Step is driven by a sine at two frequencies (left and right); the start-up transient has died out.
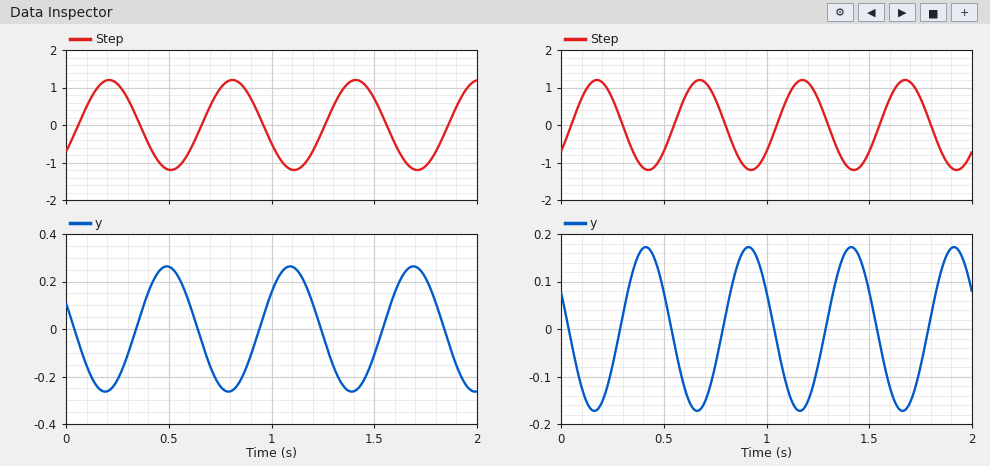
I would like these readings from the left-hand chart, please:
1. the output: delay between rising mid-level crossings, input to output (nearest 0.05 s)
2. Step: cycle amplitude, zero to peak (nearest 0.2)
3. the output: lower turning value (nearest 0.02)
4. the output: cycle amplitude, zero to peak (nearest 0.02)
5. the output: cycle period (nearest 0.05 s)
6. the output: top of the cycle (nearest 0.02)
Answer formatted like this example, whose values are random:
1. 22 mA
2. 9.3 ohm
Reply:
1. 0.30 s
2. 1.2
3. -0.26
4. 0.26
5. 0.60 s
6. 0.26
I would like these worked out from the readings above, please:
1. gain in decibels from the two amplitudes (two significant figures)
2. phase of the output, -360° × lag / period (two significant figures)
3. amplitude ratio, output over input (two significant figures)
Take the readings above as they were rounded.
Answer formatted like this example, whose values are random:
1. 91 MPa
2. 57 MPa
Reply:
1. -13 dB
2. -180°
3. 0.22
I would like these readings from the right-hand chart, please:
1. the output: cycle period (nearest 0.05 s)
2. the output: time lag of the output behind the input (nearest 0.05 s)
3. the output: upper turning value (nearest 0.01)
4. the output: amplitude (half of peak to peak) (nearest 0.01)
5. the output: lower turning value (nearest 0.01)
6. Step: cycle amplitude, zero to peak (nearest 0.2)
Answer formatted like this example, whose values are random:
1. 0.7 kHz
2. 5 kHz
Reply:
1. 0.50 s
2. 0.25 s
3. 0.17
4. 0.17
5. -0.17
6. 1.2
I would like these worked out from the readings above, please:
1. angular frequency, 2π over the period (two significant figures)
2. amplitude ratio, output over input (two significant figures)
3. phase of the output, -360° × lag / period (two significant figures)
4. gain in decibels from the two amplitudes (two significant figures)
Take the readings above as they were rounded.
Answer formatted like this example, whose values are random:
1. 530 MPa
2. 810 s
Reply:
1. 13 rad/s
2. 0.14
3. -180°
4. -17 dB
